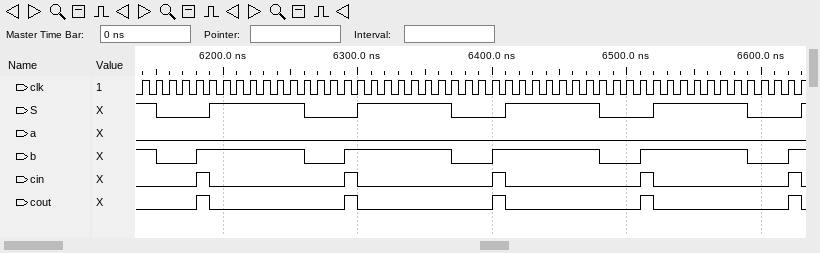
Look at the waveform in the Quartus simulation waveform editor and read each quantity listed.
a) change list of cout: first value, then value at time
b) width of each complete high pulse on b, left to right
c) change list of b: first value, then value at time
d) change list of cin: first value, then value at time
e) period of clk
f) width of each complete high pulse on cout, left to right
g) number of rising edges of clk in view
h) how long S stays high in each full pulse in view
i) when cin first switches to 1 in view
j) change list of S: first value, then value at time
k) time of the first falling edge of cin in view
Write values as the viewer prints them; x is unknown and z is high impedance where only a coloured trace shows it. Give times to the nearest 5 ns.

0, 1 at 6180 ns, 0 at 6190 ns, 1 at 6290 ns, 0 at 6300 ns, 1 at 6400 ns, 0 at 6410 ns, 1 at 6510 ns, 0 at 6520 ns, 1 at 6620 ns, 0 at 6630 ns
80 ns, 80 ns, 80 ns, 80 ns
1, 0 at 6150 ns, 1 at 6180 ns, 0 at 6260 ns, 1 at 6290 ns, 0 at 6370 ns, 1 at 6400 ns, 0 at 6480 ns, 1 at 6510 ns, 0 at 6590 ns, 1 at 6620 ns
0, 1 at 6180 ns, 0 at 6190 ns, 1 at 6290 ns, 0 at 6300 ns, 1 at 6400 ns, 0 at 6410 ns, 1 at 6510 ns, 0 at 6520 ns, 1 at 6620 ns, 0 at 6630 ns
10 ns
10 ns, 10 ns, 10 ns, 10 ns, 10 ns
50
70 ns, 70 ns, 70 ns, 70 ns
6180 ns
1, 0 at 6150 ns, 1 at 6190 ns, 0 at 6260 ns, 1 at 6300 ns, 0 at 6370 ns, 1 at 6410 ns, 0 at 6480 ns, 1 at 6520 ns, 0 at 6590 ns, 1 at 6630 ns
6190 ns
